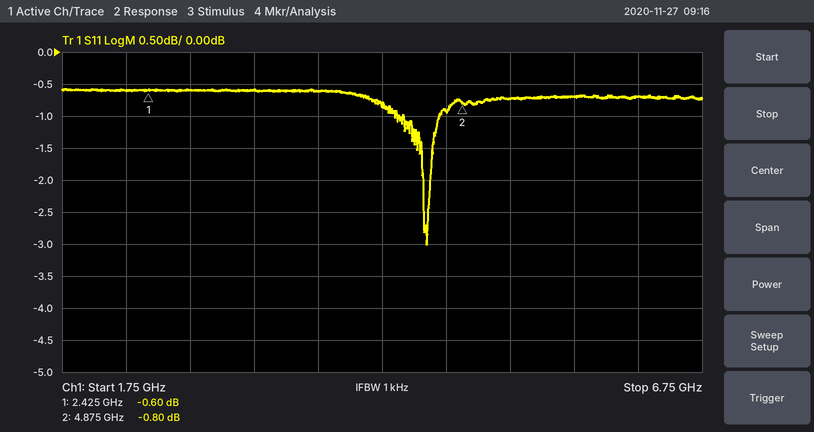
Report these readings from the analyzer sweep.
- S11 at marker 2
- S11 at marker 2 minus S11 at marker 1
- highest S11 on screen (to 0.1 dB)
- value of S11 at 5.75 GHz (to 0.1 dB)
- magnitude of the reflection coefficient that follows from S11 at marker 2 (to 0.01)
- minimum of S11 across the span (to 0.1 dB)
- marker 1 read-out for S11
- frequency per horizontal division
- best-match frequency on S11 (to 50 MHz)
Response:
-0.80 dB
-0.20 dB
-0.6 dB
-0.7 dB
0.91
-3.0 dB
-0.60 dB
500 MHz
4.60 GHz
